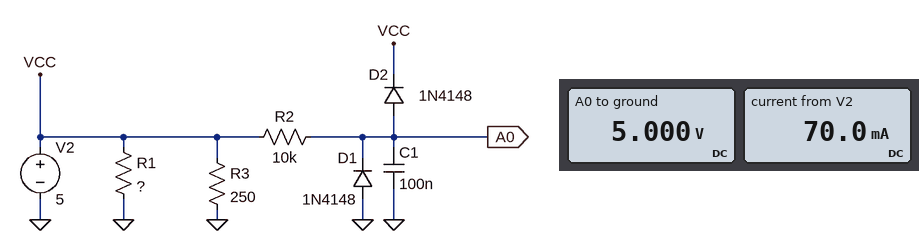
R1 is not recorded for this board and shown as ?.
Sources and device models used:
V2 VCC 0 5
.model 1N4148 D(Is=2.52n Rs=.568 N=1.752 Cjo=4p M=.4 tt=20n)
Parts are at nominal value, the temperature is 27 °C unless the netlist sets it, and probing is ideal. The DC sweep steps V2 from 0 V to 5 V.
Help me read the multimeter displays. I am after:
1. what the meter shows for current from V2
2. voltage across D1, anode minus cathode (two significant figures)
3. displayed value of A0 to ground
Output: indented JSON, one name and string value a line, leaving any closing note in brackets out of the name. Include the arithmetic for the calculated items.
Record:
{
  "what the meter shows for current from V2": "70.0 mA",
  "voltage across D1, anode minus cathode": "0 V - 5 V = -5.0 V",
  "displayed value of A0 to ground": "5.000 V"
}
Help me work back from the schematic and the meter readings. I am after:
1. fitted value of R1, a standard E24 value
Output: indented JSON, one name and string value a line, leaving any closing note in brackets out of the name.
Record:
{
  "fitted value of R1, a standard E24 value": "100 Ω"
}
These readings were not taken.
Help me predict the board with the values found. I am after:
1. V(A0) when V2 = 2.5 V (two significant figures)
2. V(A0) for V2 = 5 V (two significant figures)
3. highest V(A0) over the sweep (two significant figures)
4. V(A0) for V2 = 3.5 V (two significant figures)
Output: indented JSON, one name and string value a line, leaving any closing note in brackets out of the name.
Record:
{
  "V(A0) when V2 = 2.5 V": "2.5 V",
  "V(A0) for V2 = 5 V": "5.0 V",
  "highest V(A0) over the sweep": "5.0 V",
  "V(A0) for V2 = 3.5 V": "3.5 V"
}
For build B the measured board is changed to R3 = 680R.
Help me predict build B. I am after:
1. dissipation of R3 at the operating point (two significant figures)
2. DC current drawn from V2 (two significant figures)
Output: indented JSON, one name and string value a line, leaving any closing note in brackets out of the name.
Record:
{
  "dissipation of R3 at the operating point": "37 mW",
  "DC current drawn from V2": "57 mA"
}
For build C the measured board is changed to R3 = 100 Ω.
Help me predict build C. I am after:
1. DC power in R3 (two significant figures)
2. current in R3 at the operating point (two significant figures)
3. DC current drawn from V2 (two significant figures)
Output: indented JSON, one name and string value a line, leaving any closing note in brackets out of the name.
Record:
{
  "DC power in R3": "250 mW",
  "current in R3 at the operating point": "50 mA",
  "DC current drawn from V2": "100 mA"
}
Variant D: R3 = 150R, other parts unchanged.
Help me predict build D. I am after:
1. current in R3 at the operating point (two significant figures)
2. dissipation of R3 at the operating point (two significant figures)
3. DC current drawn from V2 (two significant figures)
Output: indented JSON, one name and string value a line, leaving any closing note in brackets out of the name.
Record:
{
  "current in R3 at the operating point": "33 mA",
  "dissipation of R3 at the operating point": "170 mW",
  "DC current drawn from V2": "83 mA"
}
